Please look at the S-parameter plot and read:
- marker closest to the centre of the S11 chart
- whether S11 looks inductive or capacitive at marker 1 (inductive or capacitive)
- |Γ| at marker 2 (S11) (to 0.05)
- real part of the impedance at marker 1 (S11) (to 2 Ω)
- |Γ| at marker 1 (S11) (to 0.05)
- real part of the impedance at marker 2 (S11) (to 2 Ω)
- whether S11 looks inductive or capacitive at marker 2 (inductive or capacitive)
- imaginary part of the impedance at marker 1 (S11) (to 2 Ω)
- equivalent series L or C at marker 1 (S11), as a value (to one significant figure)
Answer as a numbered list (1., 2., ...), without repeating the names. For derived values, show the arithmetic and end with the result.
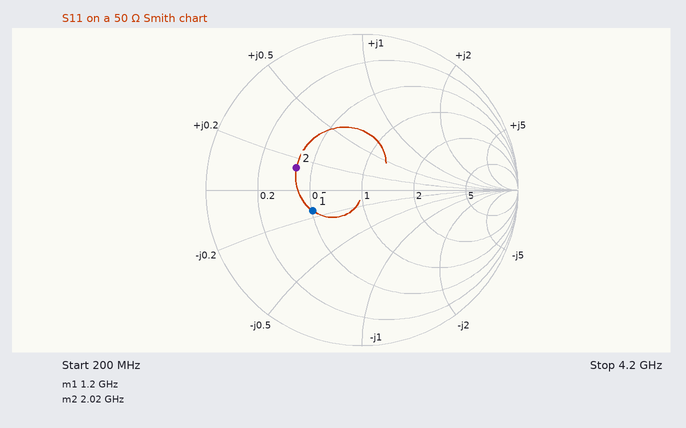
1. marker 1
2. capacitive
3. 0.45
4. 26 Ω
5. 0.35
6. 20 Ω
7. inductive
8. -8 Ω
9. C = 1/(2π × 1.2 GHz × 8 Ω) ≈ 16.6 pF, so 20 pF to one significant figure
